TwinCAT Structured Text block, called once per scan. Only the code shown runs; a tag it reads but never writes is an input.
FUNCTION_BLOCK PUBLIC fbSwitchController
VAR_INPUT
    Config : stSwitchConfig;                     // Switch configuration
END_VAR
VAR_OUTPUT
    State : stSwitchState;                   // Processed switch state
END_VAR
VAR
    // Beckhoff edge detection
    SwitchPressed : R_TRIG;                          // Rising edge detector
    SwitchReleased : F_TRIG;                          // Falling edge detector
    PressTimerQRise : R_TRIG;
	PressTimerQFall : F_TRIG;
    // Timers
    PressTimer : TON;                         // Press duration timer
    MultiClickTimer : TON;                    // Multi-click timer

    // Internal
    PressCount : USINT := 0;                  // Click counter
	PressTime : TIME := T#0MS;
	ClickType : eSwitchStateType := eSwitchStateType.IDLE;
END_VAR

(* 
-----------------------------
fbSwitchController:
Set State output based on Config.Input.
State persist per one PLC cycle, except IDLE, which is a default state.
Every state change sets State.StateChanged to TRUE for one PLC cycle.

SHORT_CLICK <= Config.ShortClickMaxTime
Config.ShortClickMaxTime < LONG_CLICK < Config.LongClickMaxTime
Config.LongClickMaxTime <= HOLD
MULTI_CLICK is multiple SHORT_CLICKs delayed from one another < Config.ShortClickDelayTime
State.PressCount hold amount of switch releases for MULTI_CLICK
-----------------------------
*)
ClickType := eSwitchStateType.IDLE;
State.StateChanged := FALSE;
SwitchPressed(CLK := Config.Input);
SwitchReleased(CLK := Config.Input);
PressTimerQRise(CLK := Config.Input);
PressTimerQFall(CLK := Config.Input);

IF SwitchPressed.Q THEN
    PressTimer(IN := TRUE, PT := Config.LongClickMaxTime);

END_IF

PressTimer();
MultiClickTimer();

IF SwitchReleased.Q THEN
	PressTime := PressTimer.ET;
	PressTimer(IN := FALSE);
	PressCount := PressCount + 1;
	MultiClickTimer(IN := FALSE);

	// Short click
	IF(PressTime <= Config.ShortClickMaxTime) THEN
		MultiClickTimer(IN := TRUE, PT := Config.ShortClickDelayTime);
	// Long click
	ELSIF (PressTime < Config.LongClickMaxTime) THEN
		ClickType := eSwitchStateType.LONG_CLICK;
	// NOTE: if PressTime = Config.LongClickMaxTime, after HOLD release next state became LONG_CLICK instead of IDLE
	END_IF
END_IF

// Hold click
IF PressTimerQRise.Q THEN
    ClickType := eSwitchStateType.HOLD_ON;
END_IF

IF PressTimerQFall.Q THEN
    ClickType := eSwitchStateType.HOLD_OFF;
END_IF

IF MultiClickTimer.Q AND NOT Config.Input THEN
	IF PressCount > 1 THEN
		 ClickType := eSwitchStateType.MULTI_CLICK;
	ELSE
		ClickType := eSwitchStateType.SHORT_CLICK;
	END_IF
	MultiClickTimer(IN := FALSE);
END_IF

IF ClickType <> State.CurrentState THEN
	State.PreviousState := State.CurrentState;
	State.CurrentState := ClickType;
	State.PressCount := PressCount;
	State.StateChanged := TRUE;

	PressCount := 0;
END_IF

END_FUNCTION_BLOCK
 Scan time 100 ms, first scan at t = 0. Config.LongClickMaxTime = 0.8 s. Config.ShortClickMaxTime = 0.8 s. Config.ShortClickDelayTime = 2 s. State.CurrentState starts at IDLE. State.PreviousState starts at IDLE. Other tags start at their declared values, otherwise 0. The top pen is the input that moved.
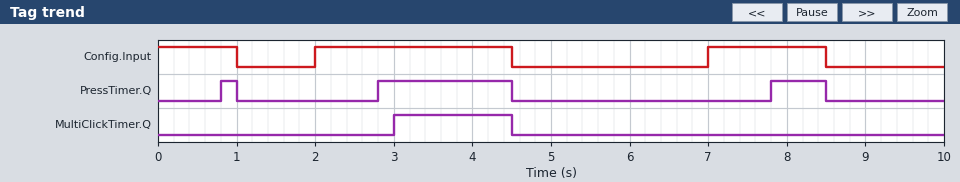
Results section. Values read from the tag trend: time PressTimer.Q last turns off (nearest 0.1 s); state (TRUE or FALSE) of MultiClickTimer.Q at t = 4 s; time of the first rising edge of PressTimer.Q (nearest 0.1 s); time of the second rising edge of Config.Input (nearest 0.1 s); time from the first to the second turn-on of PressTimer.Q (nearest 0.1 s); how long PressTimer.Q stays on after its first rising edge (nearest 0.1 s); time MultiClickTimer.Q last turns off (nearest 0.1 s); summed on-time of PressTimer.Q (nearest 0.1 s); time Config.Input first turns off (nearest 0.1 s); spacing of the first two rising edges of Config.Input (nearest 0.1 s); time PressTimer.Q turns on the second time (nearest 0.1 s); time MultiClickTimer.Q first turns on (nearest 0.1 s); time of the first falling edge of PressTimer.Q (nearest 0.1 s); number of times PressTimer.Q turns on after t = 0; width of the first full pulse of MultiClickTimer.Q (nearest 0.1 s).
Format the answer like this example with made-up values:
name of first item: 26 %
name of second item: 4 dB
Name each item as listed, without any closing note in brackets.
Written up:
time PressTimer.Q last turns off: 8.5 s
state (TRUE or FALSE) of MultiClickTimer.Q at t = 4 s: TRUE
time of the first rising edge of PressTimer.Q: 0.8 s
time of the second rising edge of Config.Input: 7.0 s
time from the first to the second turn-on of PressTimer.Q: 2.0 s
how long PressTimer.Q stays on after its first rising edge: 0.2 s
time MultiClickTimer.Q last turns off: 4.5 s
summed on-time of PressTimer.Q: 2.6 s
time Config.Input first turns off: 1.0 s
spacing of the first two rising edges of Config.Input: 5.0 s
time PressTimer.Q turns on the second time: 2.8 s
time MultiClickTimer.Q first turns on: 3.0 s
time of the first falling edge of PressTimer.Q: 1.0 s
number of times PressTimer.Q turns on after t = 0: 3
width of the first full pulse of MultiClickTimer.Q: 1.5 s
